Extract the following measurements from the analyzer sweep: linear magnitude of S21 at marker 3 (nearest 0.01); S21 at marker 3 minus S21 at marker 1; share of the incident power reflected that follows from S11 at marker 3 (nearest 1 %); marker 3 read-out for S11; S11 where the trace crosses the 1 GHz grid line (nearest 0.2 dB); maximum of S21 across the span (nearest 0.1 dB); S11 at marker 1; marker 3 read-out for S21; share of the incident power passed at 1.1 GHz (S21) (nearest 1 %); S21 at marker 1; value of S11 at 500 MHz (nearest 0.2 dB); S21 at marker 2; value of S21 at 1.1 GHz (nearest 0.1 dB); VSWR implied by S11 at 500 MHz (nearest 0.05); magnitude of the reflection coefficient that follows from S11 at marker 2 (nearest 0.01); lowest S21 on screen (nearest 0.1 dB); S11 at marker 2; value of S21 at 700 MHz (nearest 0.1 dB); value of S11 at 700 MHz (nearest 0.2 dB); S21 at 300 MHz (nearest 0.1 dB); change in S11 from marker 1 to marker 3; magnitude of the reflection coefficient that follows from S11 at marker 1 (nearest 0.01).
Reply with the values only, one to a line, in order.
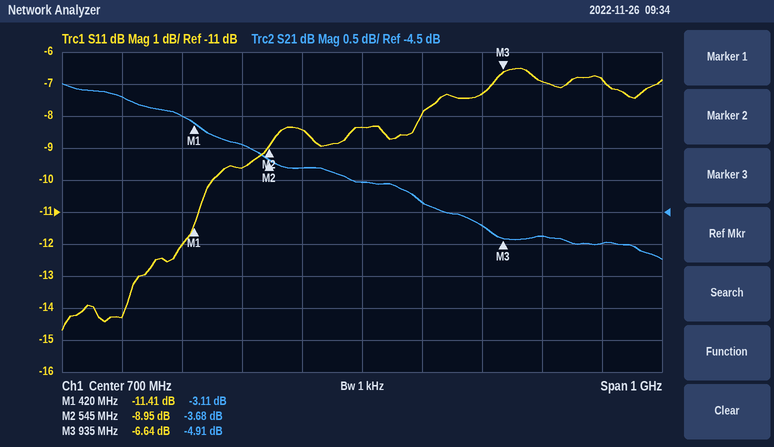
0.57
-1.80 dB
22 %
-6.64 dB
-7.0 dB
-2.5 dB
-11.41 dB
-4.91 dB
32 %
-3.11 dB
-9.6 dB
-3.68 dB
-5.0 dB
2.00
0.36
-5.2 dB
-8.95 dB
-4.0 dB
-8.4 dB
-2.7 dB
4.77 dB
0.27
